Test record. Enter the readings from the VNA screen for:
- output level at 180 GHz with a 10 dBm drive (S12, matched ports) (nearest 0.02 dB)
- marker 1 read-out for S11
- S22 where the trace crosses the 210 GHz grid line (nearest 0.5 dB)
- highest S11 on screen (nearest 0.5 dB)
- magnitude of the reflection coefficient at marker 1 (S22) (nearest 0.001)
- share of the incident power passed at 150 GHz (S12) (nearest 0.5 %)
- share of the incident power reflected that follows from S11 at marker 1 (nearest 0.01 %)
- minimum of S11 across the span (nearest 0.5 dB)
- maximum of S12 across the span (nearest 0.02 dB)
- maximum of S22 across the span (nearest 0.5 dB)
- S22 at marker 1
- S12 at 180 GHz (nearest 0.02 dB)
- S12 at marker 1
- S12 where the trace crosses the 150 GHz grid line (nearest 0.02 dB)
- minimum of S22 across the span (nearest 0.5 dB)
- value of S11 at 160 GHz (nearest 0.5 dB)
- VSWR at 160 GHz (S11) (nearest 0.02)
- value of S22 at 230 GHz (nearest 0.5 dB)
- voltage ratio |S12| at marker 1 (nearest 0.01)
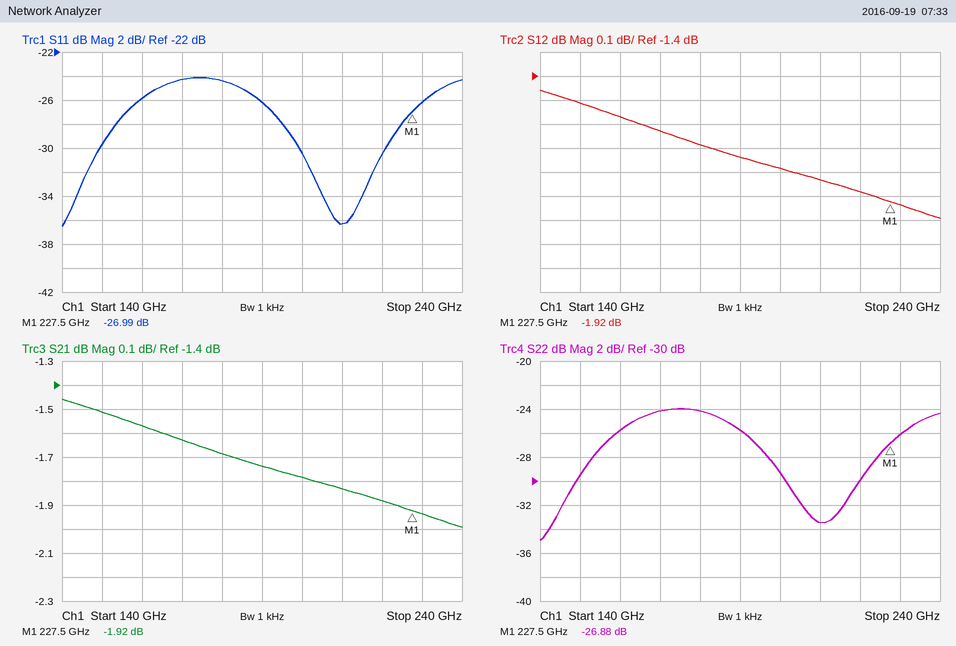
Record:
8.32 dBm
-26.99 dB
-33.5 dB
-24.0 dB
0.045
70.5 %
0.20 %
-36.5 dB
-1.46 dB
-24.0 dB
-26.88 dB
-1.68 dB
-1.92 dB
-1.52 dB
-35.0 dB
-26.0 dB
1.10
-26.0 dB
0.80
